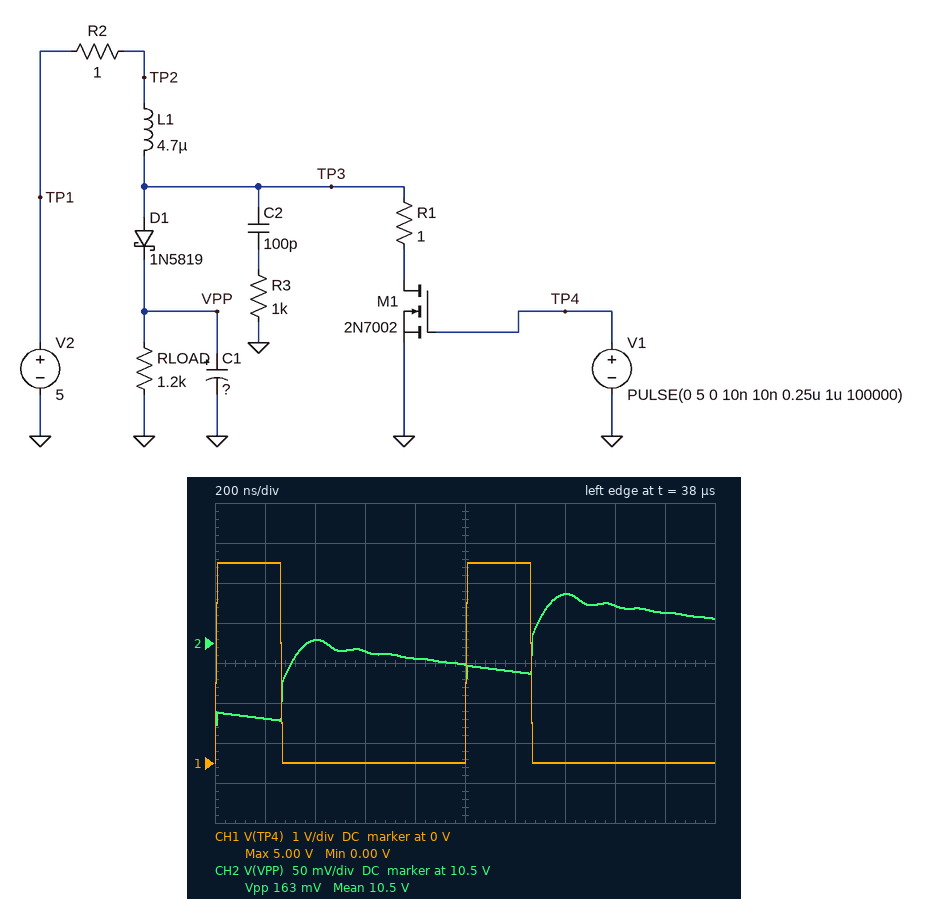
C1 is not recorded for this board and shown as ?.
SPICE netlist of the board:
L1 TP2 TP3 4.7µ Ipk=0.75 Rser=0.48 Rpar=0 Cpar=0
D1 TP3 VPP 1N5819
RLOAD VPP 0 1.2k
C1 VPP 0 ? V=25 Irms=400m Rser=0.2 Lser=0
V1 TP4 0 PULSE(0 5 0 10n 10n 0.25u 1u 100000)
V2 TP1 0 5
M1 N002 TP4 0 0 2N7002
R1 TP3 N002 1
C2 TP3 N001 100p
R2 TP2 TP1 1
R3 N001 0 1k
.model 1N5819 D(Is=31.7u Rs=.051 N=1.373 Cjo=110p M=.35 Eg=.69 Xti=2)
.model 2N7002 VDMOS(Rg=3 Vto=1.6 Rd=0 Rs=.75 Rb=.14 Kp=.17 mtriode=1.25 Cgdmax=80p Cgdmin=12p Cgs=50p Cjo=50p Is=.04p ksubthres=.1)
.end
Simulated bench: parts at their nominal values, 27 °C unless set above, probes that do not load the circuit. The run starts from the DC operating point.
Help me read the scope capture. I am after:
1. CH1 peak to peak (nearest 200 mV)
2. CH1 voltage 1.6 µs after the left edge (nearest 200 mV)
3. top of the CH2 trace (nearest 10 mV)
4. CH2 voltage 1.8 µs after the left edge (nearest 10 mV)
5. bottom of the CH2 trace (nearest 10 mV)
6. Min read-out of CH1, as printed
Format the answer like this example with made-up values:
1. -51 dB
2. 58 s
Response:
1. 5.0 V
2. 0 V
3. 10.56 V
4. 10.54 V
5. 10.40 V
6. 0.00 V
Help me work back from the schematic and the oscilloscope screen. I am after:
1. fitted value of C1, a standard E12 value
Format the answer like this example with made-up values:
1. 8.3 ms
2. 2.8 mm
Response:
1. 220 nF
